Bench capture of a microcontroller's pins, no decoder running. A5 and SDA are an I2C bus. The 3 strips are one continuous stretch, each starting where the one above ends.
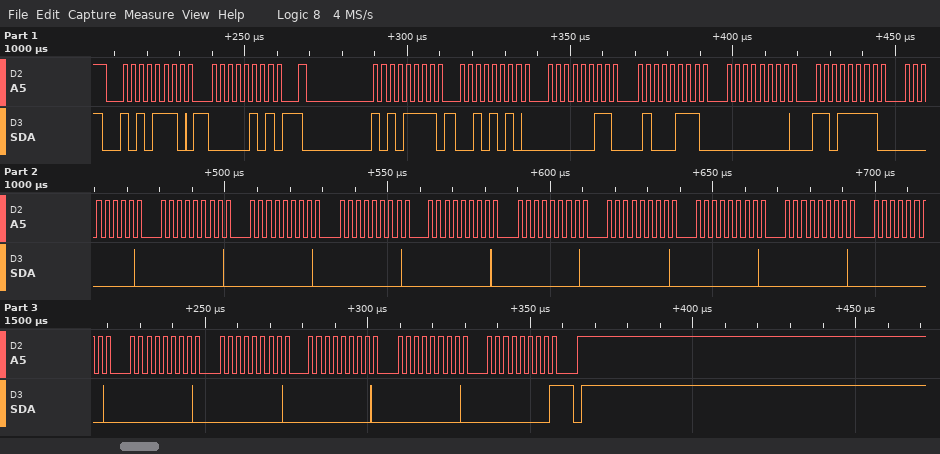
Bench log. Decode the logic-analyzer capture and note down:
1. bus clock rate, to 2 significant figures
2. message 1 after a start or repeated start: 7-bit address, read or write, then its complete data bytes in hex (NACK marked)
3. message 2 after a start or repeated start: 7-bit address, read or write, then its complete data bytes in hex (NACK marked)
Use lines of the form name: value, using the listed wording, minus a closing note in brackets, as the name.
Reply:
bus clock rate, to 2 significant figures: 400 kHz
message 1 after a start or repeated start: 7-bit address, read or write, then its complete data bytes in hex: 0x57 write: 05
message 2 after a start or repeated start: 7-bit address, read or write, then its complete data bytes in hex: 0x57 read: 2A 03 47 00 DF 00 00 00 00 00 00 00 00 00 00 00 00 00 00 00 NACK
